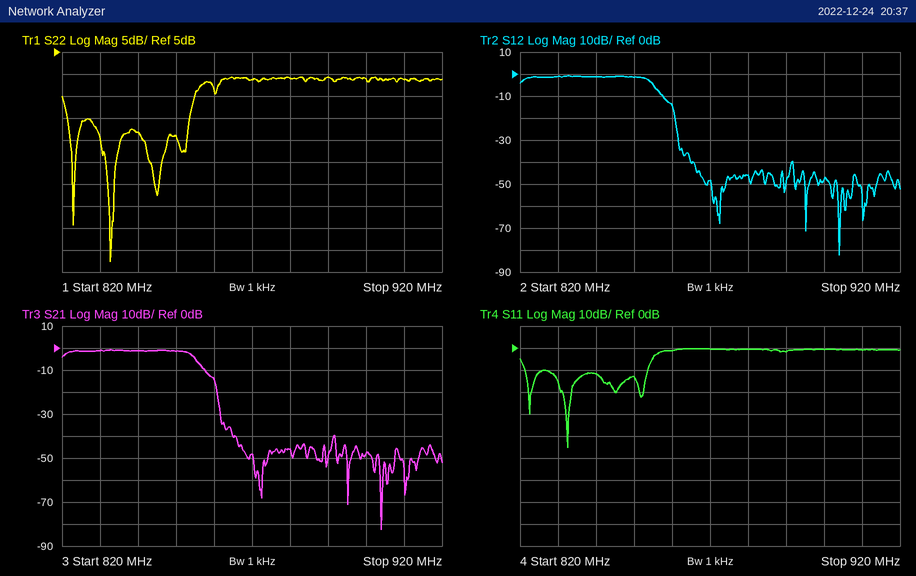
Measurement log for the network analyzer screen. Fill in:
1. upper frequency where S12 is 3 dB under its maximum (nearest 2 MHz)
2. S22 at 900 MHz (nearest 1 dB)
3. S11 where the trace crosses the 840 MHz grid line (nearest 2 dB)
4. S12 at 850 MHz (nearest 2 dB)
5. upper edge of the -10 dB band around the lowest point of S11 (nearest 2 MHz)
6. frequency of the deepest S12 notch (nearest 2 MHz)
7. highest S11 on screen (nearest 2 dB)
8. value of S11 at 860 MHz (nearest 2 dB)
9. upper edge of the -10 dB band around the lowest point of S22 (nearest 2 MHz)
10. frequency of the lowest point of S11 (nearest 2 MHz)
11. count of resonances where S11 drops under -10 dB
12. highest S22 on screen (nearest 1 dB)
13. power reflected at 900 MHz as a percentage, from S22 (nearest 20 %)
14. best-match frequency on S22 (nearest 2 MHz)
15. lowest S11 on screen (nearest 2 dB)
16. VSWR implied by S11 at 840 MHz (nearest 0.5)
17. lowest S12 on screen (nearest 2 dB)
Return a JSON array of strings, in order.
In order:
["854 MHz", "-1 dB", "-12 dB", "-2 dB", "854 MHz", "904 MHz", "0 dB", "-2 dB", "854 MHz", "832 MHz", "4", "-1 dB", "80 %", "832 MHz", "-46 dB", "1.5", "-82 dB"]
